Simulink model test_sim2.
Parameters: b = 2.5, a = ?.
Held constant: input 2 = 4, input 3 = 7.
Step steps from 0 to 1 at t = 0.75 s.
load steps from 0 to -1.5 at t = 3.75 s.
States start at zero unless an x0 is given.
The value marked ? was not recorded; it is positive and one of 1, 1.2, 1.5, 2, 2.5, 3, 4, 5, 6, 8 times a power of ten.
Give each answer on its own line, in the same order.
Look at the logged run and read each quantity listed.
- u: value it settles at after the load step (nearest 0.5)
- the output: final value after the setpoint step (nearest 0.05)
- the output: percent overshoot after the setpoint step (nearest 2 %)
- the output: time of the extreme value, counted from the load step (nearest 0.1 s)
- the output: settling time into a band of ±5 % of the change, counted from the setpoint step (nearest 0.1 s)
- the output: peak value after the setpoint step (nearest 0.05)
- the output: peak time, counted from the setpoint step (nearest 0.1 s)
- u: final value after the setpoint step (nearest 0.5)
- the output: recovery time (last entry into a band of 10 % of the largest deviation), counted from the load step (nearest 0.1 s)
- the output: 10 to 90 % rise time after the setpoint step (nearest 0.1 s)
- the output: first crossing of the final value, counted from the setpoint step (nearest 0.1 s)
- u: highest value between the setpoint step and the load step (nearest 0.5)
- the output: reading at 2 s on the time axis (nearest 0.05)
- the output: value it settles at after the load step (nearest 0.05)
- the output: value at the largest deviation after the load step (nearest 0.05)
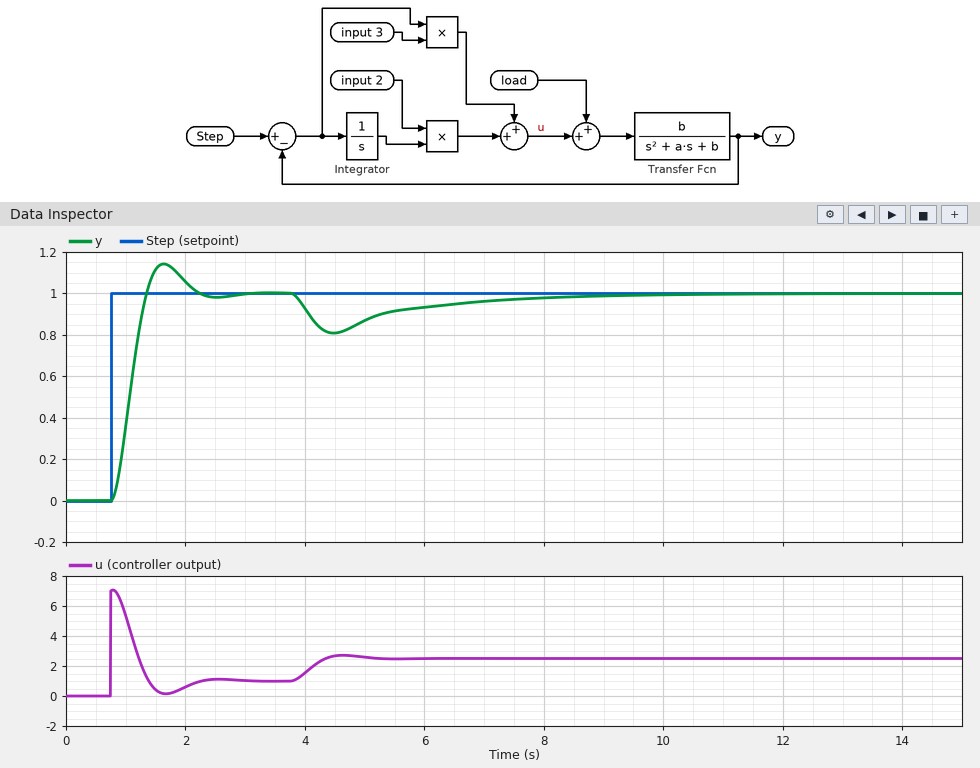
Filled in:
2.5
1.00
14 %
0.7 s
1.3 s
1.15
0.9 s
1.0
4.4 s
0.4 s
0.6 s
7.0
1.05
1.00
0.80
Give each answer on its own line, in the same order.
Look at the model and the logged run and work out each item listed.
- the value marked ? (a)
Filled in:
5
